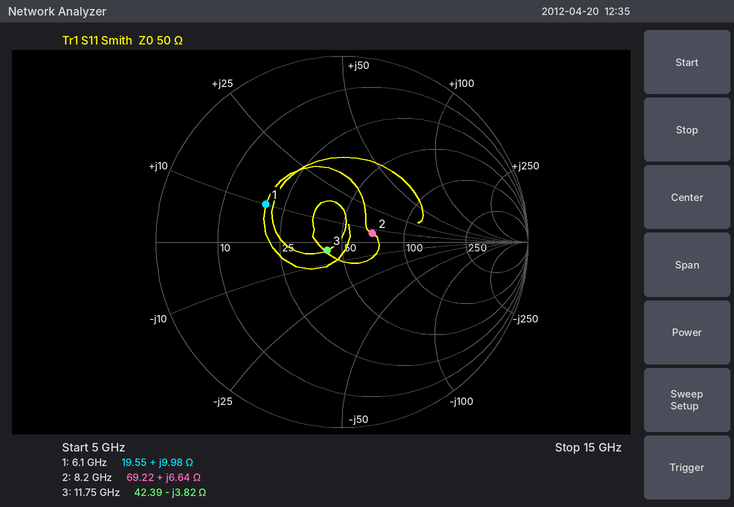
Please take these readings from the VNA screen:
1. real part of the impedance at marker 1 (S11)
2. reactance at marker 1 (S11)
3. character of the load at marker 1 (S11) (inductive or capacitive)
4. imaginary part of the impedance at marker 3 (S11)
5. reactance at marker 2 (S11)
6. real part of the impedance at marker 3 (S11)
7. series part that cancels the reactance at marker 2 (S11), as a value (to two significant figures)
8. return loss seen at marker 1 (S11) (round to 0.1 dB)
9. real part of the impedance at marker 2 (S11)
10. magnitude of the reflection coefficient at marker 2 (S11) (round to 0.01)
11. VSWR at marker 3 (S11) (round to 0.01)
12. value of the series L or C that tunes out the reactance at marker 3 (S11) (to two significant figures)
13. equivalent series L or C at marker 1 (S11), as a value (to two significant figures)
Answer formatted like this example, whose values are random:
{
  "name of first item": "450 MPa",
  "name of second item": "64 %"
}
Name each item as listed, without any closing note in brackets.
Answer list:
{
  "real part of the impedance at marker 1": "19.55 Ω",
  "reactance at marker 1": "+9.98 Ω",
  "character of the load at marker 1 (S11)": "inductive",
  "imaginary part of the impedance at marker 3": "-3.82 Ω",
  "reactance at marker 2": "+6.64 Ω",
  "real part of the impedance at marker 3": "42.39 Ω",
  "series part that cancels the reactance at marker 2 (S11), as a value": "2.9 pF",
  "return loss seen at marker 1 (S11)": "6.8 dB",
  "real part of the impedance at marker 2": "69.22 Ω",
  "magnitude of the reflection coefficient at marker 2 (S11)": "0.17",
  "VSWR at marker 3 (S11)": "1.20",
  "value of the series L or C that tunes out the reactance at marker 3 (S11)": "52 pH",
  "equivalent series L or C at marker 1 (S11), as a value": "260 pH"
}
